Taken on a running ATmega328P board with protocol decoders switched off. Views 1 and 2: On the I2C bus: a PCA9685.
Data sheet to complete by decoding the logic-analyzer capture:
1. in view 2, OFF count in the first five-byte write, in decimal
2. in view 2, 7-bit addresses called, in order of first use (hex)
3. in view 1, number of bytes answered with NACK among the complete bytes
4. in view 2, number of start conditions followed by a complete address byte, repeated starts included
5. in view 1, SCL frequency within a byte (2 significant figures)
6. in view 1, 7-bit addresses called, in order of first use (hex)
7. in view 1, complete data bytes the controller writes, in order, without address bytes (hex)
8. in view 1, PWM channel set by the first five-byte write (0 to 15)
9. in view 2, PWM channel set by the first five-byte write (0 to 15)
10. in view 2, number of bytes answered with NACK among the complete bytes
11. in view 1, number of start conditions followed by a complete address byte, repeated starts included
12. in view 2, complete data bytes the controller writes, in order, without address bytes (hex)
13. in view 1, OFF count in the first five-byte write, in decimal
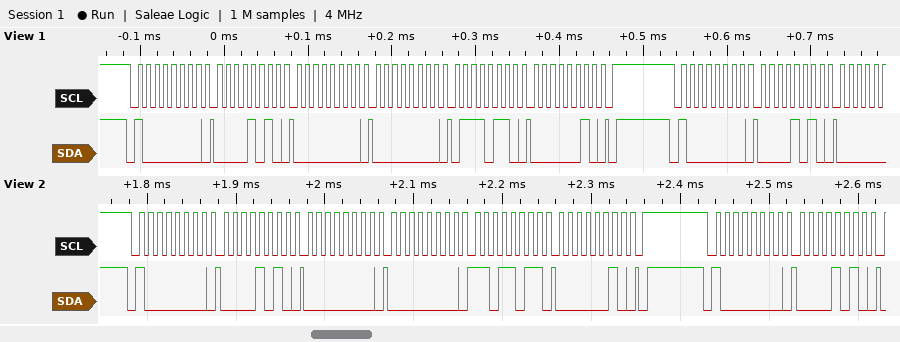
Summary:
731
0x40
0
2
100 kHz
0x40
0A 00 00 76 02 0A
1
1
0
2
0A 00 00 DB 02 0A
630
